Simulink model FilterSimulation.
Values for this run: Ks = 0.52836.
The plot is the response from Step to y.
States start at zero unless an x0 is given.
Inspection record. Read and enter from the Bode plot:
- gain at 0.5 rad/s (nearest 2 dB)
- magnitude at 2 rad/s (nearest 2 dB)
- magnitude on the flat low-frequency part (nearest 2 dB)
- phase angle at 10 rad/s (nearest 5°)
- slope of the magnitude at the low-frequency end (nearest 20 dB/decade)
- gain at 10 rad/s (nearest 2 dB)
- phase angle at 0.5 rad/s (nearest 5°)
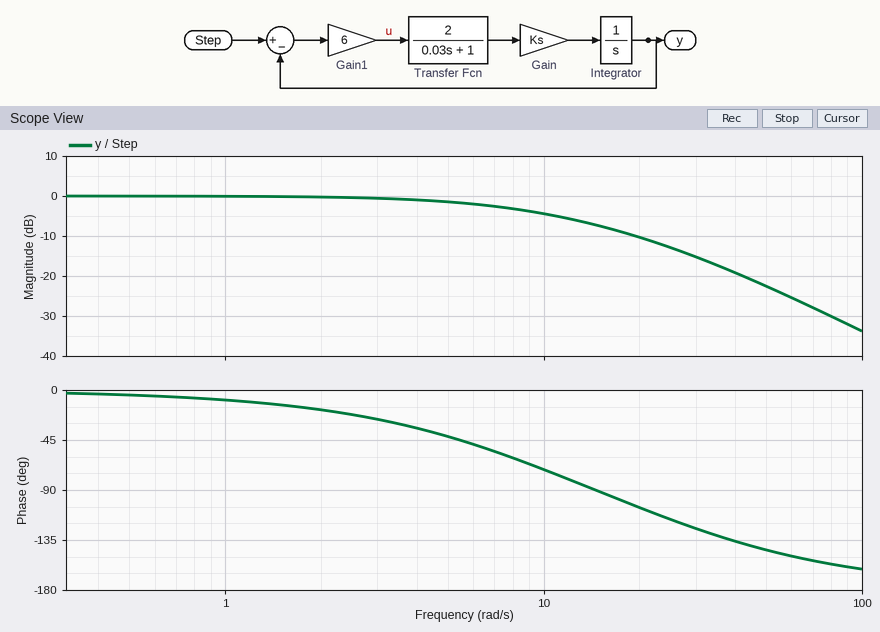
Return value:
0 dB
0 dB
0 dB
-70°
0 dB/decade
-4 dB
-5°
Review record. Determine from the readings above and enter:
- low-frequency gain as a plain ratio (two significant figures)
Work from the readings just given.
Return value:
1.0
